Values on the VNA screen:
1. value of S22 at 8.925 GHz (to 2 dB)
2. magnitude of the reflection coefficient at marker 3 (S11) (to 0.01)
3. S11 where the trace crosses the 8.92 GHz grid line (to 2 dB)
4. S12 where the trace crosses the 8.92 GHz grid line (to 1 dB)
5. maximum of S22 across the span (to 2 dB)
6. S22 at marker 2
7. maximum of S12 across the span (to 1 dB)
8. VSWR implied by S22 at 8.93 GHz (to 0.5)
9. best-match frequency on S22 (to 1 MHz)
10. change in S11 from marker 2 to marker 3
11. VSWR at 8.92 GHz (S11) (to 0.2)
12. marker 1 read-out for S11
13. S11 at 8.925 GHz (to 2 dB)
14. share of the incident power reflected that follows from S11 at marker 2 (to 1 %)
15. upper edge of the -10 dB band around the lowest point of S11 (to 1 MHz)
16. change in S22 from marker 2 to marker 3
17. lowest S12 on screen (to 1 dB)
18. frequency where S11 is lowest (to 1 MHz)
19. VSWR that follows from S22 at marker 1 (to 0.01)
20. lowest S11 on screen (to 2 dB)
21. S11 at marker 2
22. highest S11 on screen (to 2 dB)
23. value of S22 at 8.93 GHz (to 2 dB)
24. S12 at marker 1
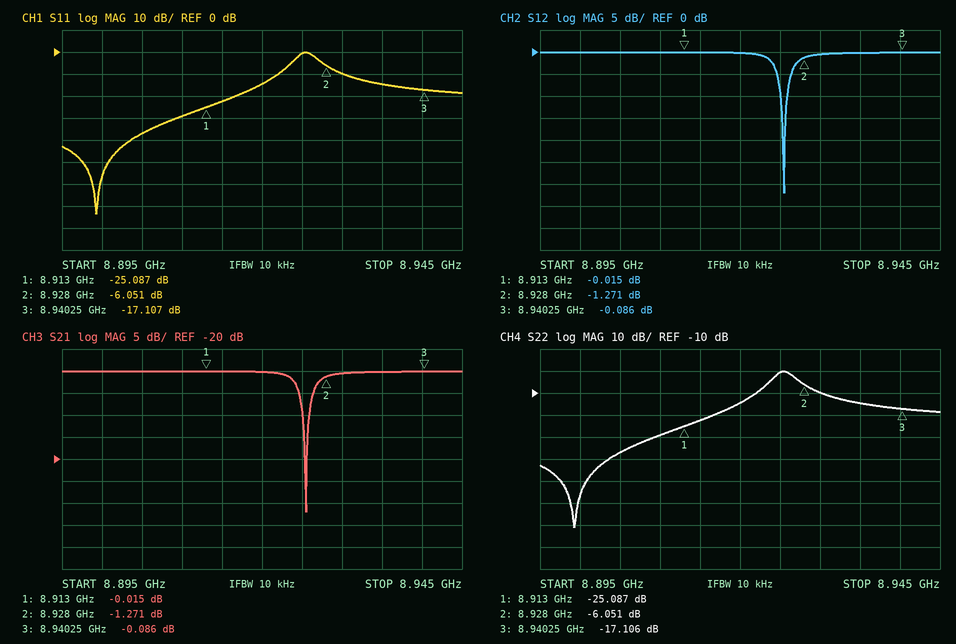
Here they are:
0 dB
0.14
-14 dB
0 dB
0 dB
-6.051 dB
0 dB
2.0
8.899 GHz
-11.056 dB
1.4
-25.087 dB
0 dB
25 %
8.922 GHz
-11.055 dB
-32 dB
8.899 GHz
1.12
-74 dB
-6.051 dB
0 dB
-10 dB
-0.015 dB
